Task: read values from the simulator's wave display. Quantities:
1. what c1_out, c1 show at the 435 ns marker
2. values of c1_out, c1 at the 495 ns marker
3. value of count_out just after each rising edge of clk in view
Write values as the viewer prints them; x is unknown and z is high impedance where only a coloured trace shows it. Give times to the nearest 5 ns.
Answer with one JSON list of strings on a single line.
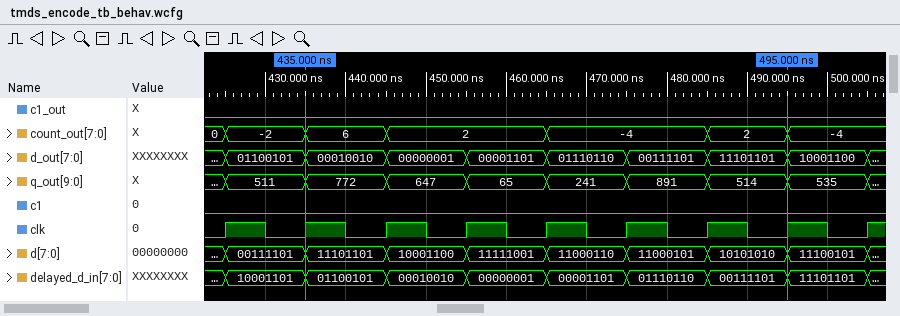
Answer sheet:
["c1_out=0, c1=0", "c1_out=0, c1=0", "-2, 6, 2, 2, -4, -4, 2, -4, -4"]
